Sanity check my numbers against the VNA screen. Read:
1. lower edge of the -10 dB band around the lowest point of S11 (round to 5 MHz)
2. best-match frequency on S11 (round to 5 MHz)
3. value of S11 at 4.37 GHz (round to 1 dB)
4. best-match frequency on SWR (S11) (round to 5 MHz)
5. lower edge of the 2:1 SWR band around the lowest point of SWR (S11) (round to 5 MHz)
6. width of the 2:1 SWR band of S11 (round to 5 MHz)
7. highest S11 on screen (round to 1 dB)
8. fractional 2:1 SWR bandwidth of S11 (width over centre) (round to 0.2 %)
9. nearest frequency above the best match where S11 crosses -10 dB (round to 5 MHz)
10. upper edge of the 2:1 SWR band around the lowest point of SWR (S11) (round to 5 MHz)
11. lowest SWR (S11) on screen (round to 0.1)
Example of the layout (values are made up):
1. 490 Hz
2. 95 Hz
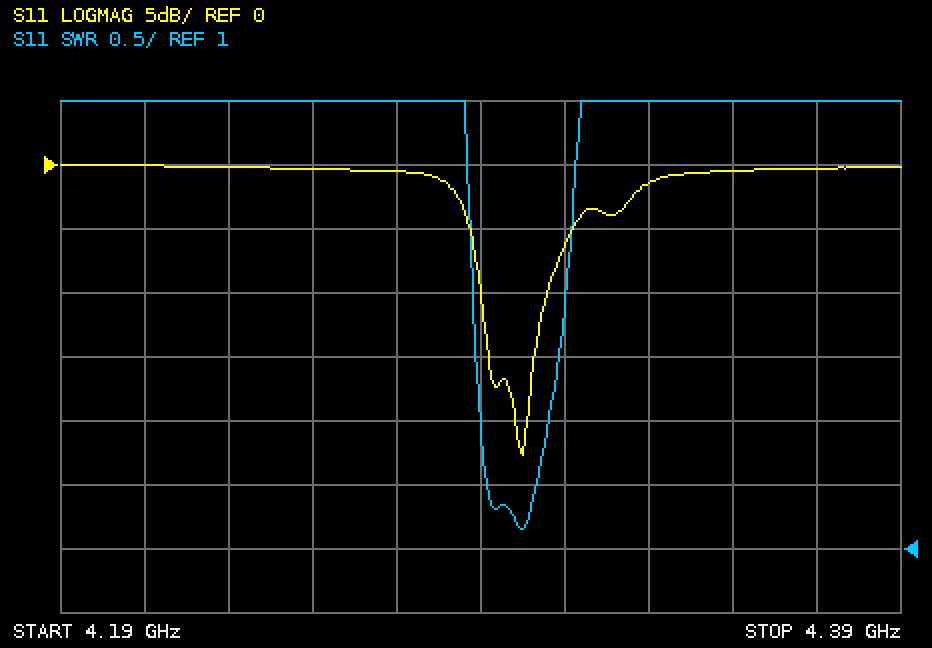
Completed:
1. 4.290 GHz
2. 4.300 GHz
3. 0 dB
4. 4.300 GHz
5. 4.290 GHz
6. 15 MHz
7. 0 dB
8. 0.4 %
9. 4.305 GHz
10. 4.305 GHz
11. 1.2
